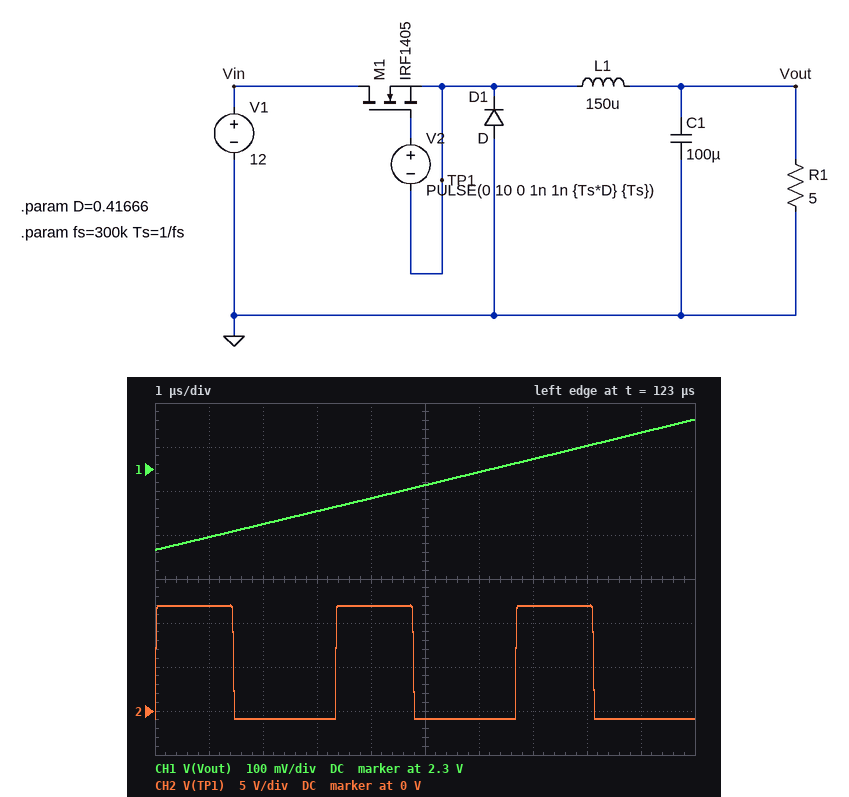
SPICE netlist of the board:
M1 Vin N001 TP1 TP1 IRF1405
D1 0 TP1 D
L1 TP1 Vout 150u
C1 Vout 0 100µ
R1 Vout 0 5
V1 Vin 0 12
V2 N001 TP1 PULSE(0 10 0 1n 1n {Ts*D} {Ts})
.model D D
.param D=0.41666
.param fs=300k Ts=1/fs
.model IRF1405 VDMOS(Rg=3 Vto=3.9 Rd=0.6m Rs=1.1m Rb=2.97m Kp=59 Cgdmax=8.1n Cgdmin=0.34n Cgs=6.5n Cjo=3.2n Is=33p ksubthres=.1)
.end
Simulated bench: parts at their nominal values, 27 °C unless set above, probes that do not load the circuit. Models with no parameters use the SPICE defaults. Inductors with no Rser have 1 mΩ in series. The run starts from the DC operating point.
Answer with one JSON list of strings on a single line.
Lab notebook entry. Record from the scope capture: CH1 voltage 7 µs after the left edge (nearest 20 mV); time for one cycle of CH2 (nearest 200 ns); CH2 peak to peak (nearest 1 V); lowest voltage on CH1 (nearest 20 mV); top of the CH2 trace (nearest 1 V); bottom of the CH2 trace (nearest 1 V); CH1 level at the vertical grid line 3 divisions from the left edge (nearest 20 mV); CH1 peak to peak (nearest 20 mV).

["2.32 V", "3.4 µs", "13 V", "2.12 V", "12 V", "-1 V", "2.20 V", "300 mV"]
